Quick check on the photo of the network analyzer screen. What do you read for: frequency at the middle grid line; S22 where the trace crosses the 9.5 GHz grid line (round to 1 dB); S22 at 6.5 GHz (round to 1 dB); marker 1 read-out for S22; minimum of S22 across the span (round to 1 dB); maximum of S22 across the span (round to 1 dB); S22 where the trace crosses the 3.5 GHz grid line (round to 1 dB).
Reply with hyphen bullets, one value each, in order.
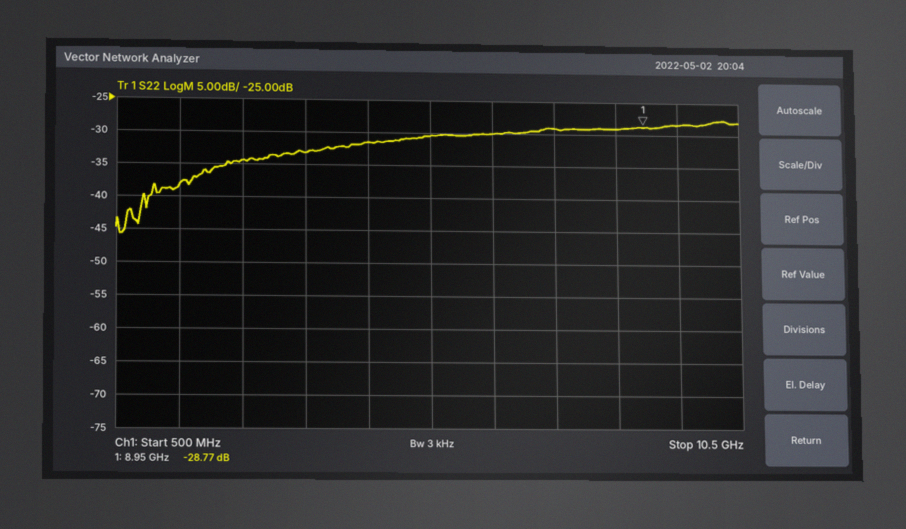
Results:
- 5.5 GHz
- -28 dB
- -30 dB
- -28.77 dB
- -46 dB
- -28 dB
- -33 dB
